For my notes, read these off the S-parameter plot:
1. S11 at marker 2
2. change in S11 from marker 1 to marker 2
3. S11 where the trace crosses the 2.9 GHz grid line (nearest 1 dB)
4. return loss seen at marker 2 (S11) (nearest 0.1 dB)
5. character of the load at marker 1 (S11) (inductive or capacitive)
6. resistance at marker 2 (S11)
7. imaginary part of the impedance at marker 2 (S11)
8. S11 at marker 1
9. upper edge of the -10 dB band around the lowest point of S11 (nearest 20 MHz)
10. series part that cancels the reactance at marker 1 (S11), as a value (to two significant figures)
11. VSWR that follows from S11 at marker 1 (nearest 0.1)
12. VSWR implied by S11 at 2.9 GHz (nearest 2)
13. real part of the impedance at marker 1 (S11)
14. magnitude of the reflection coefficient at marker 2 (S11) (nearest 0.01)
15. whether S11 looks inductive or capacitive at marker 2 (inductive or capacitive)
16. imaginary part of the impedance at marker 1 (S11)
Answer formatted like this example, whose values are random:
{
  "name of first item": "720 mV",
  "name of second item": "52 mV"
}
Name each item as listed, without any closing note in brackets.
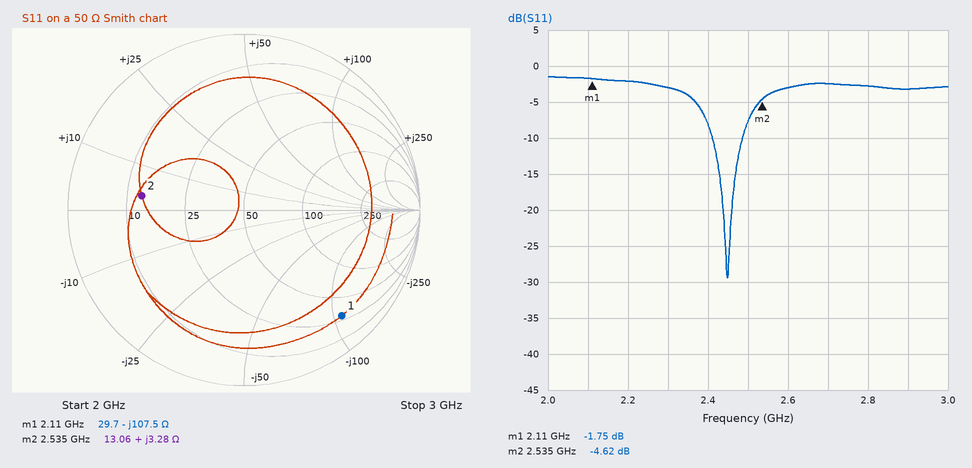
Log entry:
{
  "S11 at marker 2": "-4.62 dB",
  "change in S11 from marker 1 to marker 2": "-2.87 dB",
  "S11 where the trace crosses the 2.9 GHz grid line": "-3 dB",
  "return loss seen at marker 2 (S11)": "4.6 dB",
  "character of the load at marker 1 (S11)": "capacitive",
  "resistance at marker 2": "13.06 Ω",
  "imaginary part of the impedance at marker 2": "+3.28 Ω",
  "S11 at marker 1": "-1.75 dB",
  "upper edge of the -10 dB band around the lowest point of S11": "2.48 GHz",
  "series part that cancels the reactance at marker 1 (S11), as a value": "8.1 nH",
  "VSWR that follows from S11 at marker 1": "10.0",
  "VSWR implied by S11 at 2.9 GHz": "6",
  "real part of the impedance at marker 1": "29.7 Ω",
  "magnitude of the reflection coefficient at marker 2 (S11)": "0.59",
  "whether S11 looks inductive or capacitive at marker 2": "inductive",
  "imaginary part of the impedance at marker 1": "-107.5 Ω"
}
